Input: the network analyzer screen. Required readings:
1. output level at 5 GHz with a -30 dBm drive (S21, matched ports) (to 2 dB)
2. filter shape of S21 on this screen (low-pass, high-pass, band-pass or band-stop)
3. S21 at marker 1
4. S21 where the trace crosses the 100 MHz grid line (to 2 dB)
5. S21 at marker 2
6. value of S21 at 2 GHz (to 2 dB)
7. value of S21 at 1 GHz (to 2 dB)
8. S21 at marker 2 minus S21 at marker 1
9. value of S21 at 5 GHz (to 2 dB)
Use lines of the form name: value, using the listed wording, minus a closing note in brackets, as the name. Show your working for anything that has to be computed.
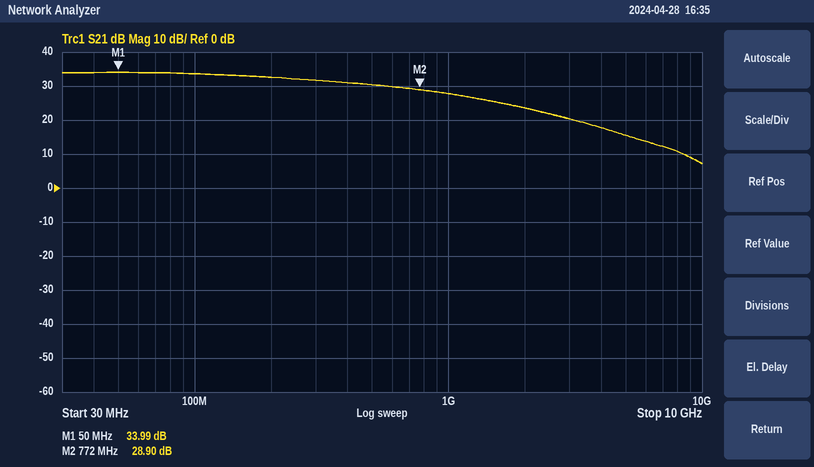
output level at 5 GHz with a -30 dBm drive (S21, matched ports): -30 dBm + (16 dB) = -14 dBm
filter shape of S21 on this screen: low-pass
S21 at marker 1: 33.99 dB
S21 where the trace crosses the 100 MHz grid line: 34 dB
S21 at marker 2: 28.90 dB
value of S21 at 2 GHz: 24 dB
value of S21 at 1 GHz: 28 dB
S21 at marker 2 minus S21 at marker 1: 28.9 − (33.99) = -5.09 dB
value of S21 at 5 GHz: 16 dB
